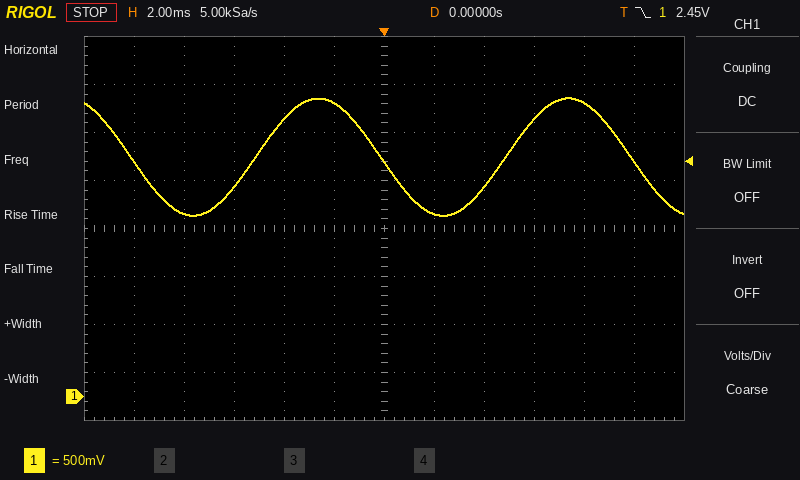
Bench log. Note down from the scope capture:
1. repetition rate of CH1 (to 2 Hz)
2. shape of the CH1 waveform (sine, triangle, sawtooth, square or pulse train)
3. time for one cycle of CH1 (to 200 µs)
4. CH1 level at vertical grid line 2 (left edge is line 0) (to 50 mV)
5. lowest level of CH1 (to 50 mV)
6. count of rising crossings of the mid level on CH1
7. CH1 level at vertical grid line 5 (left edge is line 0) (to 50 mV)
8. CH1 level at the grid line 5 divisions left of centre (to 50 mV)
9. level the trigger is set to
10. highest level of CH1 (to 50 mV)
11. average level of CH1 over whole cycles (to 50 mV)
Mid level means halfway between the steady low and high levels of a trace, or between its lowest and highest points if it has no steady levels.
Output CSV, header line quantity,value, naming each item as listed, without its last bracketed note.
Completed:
quantity,value
repetition rate of CH1,100 Hz
shape of the CH1 waveform,sine
time for one cycle of CH1,10.0 ms
CH1 level at vertical grid line 2 (left edge is line 0),1.90 V
lowest level of CH1,1.90 V
count of rising crossings of the mid level on CH1,2
CH1 level at vertical grid line 5 (left edge is line 0),3.05 V
CH1 level at the grid line 5 divisions left of centre,2.45 V
level the trigger is set to,2.45 V
highest level of CH1,3.10 V
average level of CH1 over whole cycles,2.50 V
